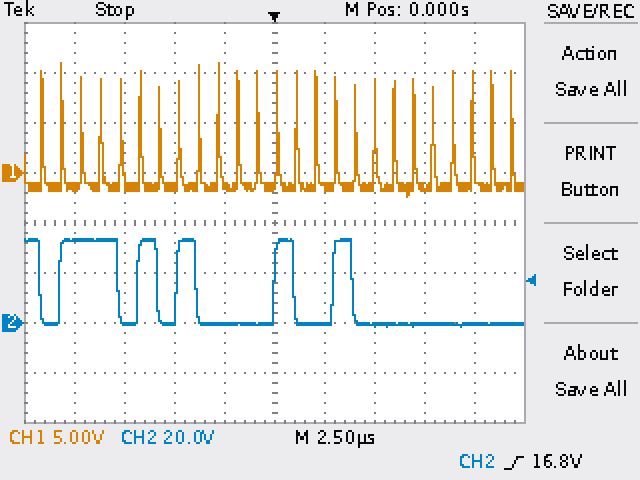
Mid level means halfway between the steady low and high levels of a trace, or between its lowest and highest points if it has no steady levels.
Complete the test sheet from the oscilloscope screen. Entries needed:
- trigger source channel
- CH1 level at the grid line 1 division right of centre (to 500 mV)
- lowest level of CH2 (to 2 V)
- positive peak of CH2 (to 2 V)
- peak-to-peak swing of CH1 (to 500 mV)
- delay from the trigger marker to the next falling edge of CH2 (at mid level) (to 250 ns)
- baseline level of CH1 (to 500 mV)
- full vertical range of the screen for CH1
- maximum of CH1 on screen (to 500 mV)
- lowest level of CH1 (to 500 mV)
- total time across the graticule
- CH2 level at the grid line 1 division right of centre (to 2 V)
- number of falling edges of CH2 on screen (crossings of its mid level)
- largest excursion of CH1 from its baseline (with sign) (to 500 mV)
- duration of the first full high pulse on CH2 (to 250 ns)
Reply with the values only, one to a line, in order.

CH2
-1.5 V
-2 V
34 V
13.5 V
1.00 µs
-1.5 V
40 V
11.0 V
-2.5 V
25 µs
0 V
6
+12.5 V
3.00 µs
